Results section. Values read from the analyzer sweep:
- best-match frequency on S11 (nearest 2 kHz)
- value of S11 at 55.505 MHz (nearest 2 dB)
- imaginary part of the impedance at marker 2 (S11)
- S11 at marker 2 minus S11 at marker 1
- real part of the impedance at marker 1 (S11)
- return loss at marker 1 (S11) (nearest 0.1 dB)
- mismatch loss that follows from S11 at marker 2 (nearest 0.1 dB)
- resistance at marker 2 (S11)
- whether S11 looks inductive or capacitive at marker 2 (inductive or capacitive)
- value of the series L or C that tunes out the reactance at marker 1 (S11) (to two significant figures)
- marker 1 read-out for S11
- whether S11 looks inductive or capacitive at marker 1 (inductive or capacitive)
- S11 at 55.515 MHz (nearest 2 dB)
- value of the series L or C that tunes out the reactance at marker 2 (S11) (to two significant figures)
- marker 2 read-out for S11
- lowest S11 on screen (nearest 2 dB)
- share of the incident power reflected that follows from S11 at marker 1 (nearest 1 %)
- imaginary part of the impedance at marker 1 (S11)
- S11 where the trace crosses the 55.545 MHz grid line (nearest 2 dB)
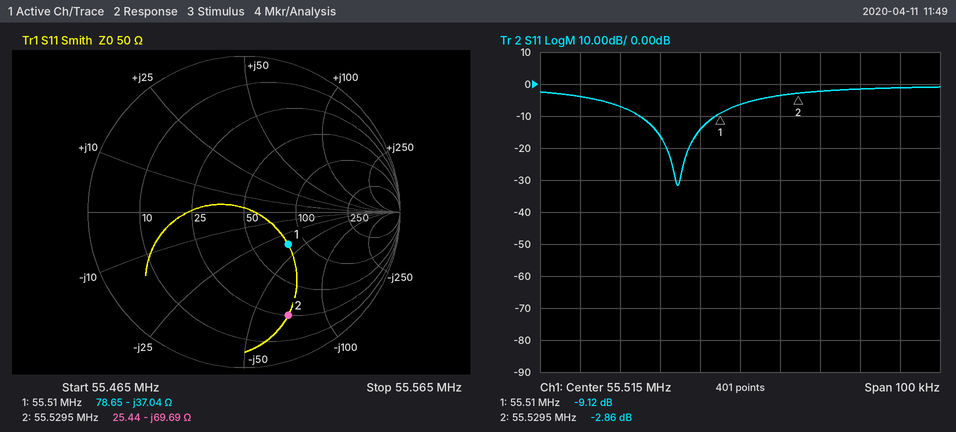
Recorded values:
55.500 MHz
-14 dB
-69.69 Ω
6.26 dB
78.65 Ω
9.1 dB
3.2 dB
25.44 Ω
capacitive
110 nH
-9.12 dB
capacitive
-6 dB
200 nH
-2.86 dB
-32 dB
12 %
-37.04 Ω
-2 dB
